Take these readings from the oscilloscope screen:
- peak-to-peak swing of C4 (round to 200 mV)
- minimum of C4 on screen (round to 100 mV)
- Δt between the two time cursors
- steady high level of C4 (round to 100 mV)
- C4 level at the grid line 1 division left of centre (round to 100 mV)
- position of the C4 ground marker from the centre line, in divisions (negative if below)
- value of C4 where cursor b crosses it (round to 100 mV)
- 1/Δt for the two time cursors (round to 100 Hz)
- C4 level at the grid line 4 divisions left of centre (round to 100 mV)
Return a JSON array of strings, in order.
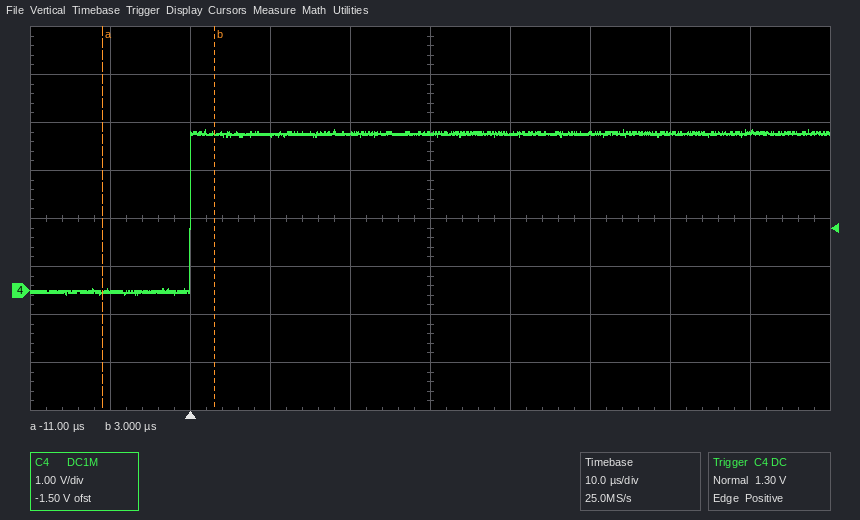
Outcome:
["3.4 V", "-100 mV", "14 µs", "3.3 V", "3.3 V", "-1.5 div", "3.3 V", "71.4 kHz", "0.0 V"]
